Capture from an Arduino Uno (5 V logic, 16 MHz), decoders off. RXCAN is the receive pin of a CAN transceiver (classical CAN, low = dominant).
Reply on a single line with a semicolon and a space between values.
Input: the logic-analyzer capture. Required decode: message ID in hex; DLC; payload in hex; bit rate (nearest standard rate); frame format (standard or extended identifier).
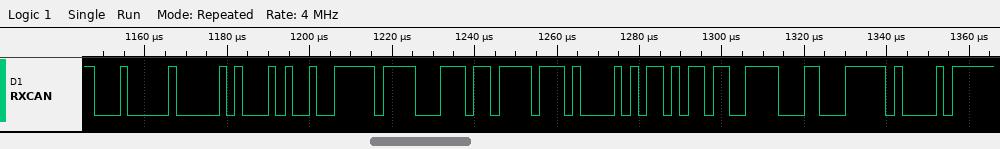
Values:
0x100; 8; A4 FF 8E DE E8 56 B6 78; 500 kbit/s; standard
